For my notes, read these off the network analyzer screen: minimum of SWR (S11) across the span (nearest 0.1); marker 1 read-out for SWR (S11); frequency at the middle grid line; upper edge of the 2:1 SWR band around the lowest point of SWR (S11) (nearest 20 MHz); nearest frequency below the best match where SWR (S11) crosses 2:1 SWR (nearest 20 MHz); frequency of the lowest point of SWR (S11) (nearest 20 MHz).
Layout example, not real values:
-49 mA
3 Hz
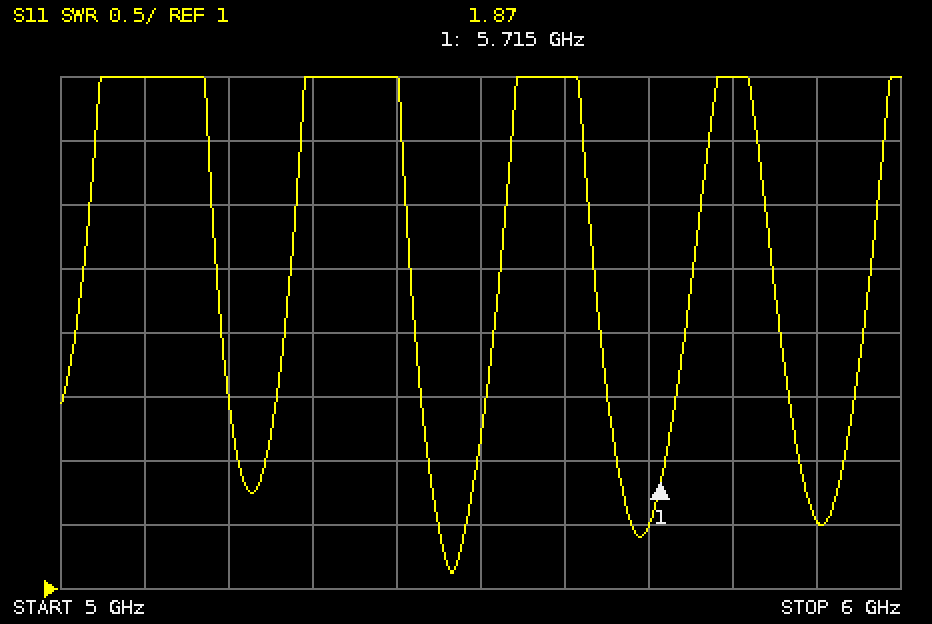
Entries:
1.1
1.87
5.5 GHz
5.50 GHz
5.44 GHz
5.46 GHz
